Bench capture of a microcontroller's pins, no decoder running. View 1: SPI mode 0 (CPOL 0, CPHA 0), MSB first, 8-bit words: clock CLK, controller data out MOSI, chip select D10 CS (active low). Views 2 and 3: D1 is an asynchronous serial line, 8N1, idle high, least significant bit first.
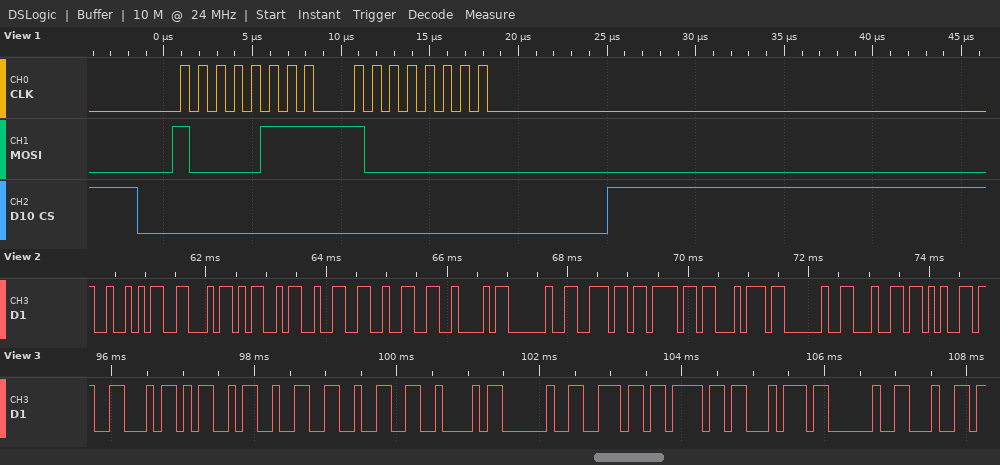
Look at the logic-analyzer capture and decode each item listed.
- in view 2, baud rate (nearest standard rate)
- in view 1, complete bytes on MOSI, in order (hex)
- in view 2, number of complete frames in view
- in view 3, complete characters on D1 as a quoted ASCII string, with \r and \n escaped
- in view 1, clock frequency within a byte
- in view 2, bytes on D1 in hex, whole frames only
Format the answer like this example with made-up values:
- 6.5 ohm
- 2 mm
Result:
- 9600 baud
- 87 80
- 13
- "FM22B not d"
- 1 MHz
- 52 46 4D 32 32 42 20 6E 6F 74 20 64 65
